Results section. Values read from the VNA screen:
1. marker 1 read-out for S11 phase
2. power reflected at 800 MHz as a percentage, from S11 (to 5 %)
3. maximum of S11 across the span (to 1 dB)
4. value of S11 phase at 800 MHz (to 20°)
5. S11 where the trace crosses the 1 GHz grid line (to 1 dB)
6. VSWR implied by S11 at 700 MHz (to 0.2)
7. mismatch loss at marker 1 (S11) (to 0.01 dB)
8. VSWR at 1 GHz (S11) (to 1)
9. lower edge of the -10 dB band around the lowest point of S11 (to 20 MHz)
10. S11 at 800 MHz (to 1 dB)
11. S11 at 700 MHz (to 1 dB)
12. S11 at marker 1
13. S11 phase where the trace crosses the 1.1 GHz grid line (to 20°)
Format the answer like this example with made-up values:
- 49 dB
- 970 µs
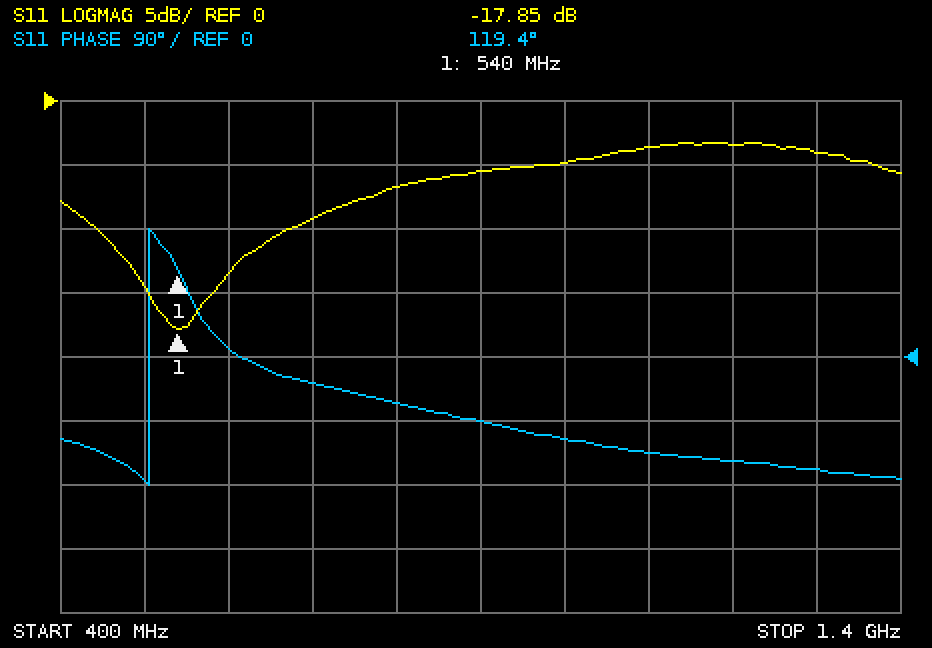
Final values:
- 119.4°
- 20 %
- -3 dB
- -60°
- -5 dB
- 2.0
- 0.07 dB
- 4
- 440 MHz
- -7 dB
- -9 dB
- -17.85 dB
- -140°
